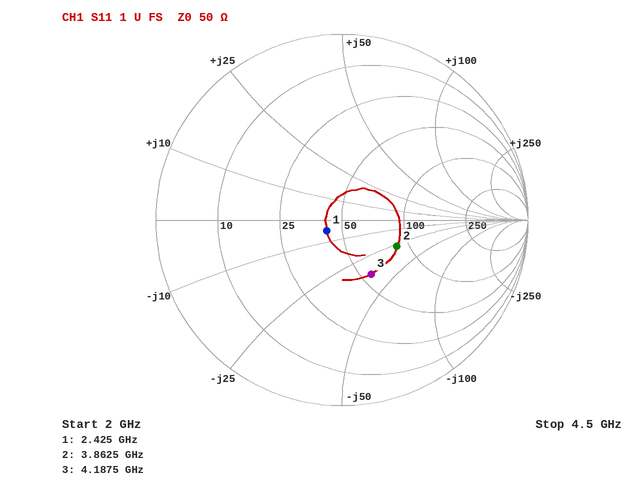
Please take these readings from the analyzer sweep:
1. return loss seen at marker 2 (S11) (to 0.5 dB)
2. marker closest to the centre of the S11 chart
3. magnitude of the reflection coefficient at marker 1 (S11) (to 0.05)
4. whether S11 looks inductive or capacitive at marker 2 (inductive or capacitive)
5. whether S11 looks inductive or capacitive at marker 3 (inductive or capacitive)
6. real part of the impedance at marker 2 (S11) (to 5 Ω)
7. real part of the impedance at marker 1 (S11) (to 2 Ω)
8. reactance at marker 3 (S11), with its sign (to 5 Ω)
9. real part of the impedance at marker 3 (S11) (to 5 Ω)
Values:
9.5 dB
marker 1
0.10
capacitive
capacitive
85 Ω
42 Ω
-35 Ω
55 Ω
